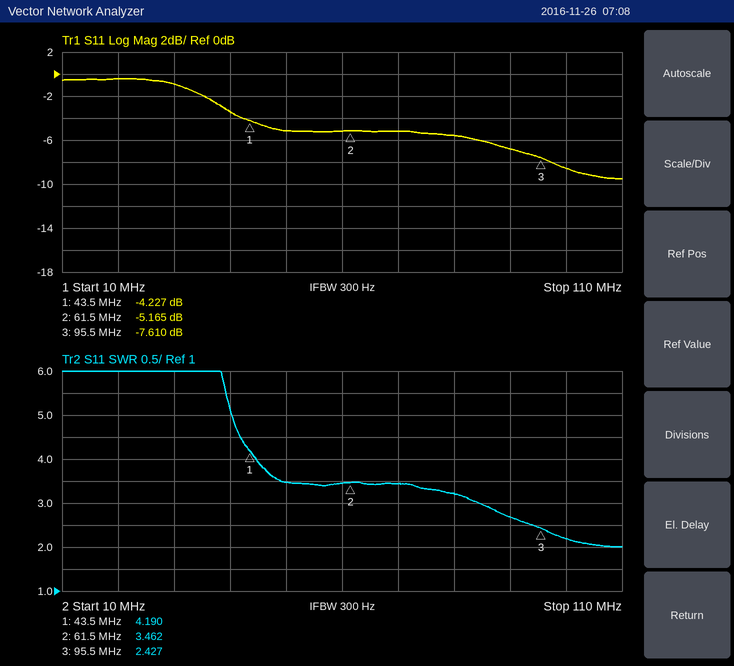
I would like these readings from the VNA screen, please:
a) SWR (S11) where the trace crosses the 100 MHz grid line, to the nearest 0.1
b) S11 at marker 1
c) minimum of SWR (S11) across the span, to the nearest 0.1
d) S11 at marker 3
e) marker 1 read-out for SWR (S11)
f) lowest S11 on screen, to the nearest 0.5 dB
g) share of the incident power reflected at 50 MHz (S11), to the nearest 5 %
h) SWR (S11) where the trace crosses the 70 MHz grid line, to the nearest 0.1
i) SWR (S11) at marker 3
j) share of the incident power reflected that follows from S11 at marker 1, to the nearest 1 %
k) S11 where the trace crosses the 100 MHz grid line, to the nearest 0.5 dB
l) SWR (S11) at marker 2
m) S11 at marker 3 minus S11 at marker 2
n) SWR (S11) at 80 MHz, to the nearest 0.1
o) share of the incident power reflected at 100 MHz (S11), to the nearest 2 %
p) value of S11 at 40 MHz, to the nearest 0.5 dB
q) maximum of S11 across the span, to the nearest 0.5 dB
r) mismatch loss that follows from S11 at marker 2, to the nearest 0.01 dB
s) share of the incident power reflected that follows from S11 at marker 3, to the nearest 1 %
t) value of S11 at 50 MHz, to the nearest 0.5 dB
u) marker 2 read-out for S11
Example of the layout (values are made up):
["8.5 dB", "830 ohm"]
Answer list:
["2.2", "-4.227 dB", "2.0", "-7.610 dB", "4.190", "-9.5 dB", "30 %", "3.4", "2.427", "38 %", "-8.5 dB", "3.462", "-2.445 dB", "3.2", "14 %", "-3.5 dB", "-0.5 dB", "1.58 dB", "17 %", "-5.0 dB", "-5.165 dB"]
